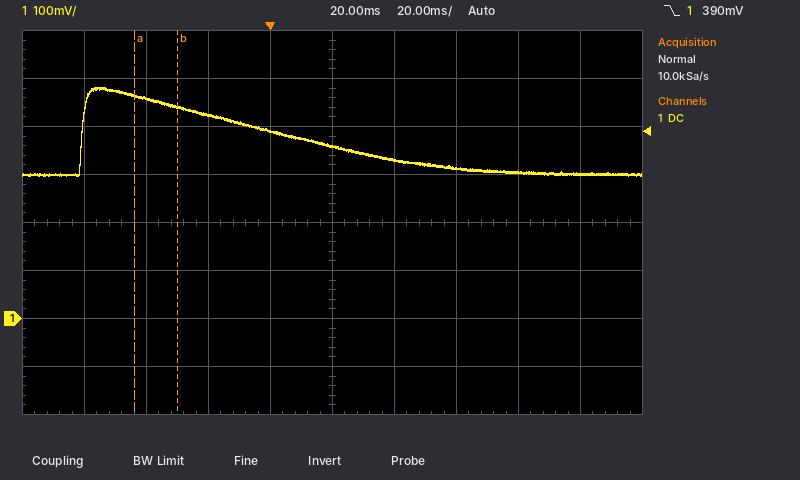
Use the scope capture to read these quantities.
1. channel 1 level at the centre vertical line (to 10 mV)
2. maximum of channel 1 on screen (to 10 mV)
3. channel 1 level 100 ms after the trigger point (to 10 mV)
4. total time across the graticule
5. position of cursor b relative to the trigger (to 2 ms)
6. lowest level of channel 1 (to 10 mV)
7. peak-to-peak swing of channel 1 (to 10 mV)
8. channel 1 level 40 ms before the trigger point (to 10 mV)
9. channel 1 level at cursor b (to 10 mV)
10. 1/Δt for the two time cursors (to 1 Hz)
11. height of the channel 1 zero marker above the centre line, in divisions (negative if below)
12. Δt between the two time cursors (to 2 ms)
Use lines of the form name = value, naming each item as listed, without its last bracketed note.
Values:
channel 1 level at the centre vertical line = 360 mV
maximum of channel 1 on screen = 480 mV
channel 1 level 100 ms after the trigger point = 300 mV
total time across the graticule = 200 ms
position of cursor b relative to the trigger = -30 ms
lowest level of channel 1 = 300 mV
peak-to-peak swing of channel 1 = 180 mV
channel 1 level 40 ms before the trigger point = 460 mV
channel 1 level at cursor b = 440 mV
1/Δt for the two time cursors = 71 Hz
height of the channel 1 zero marker above the centre line, in divisions = -2.0 div
Δt between the two time cursors = 14 ms
